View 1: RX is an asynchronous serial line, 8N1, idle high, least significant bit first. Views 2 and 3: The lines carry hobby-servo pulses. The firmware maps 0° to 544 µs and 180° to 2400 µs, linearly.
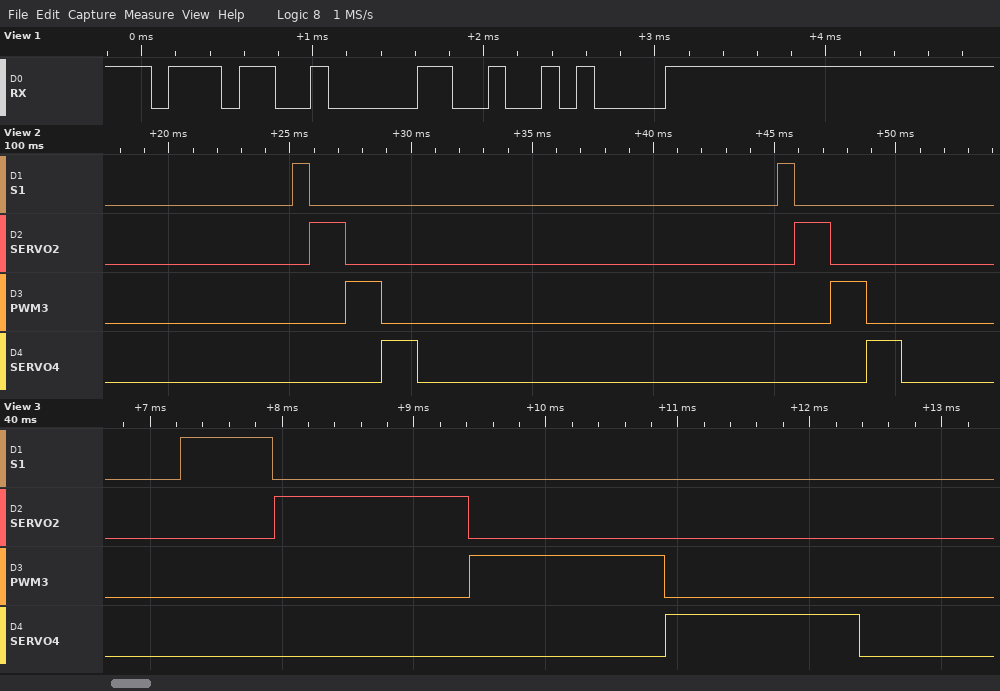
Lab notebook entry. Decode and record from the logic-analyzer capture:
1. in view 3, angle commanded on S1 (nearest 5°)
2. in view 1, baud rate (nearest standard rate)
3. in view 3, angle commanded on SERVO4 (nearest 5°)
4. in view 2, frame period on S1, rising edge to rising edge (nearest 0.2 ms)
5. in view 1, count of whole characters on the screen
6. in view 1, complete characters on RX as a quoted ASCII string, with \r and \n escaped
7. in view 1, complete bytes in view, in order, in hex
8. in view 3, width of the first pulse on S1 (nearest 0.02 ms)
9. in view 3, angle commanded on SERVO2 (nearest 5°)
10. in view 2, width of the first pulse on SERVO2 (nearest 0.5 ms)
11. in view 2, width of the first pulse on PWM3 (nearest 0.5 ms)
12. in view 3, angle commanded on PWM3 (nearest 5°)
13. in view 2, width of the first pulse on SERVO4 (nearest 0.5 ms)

15°
9600 baud
90°
20.0 ms
3
"70\n"
37 30 0A
0.70 ms
90°
1.5 ms
1.5 ms
90°
1.5 ms
